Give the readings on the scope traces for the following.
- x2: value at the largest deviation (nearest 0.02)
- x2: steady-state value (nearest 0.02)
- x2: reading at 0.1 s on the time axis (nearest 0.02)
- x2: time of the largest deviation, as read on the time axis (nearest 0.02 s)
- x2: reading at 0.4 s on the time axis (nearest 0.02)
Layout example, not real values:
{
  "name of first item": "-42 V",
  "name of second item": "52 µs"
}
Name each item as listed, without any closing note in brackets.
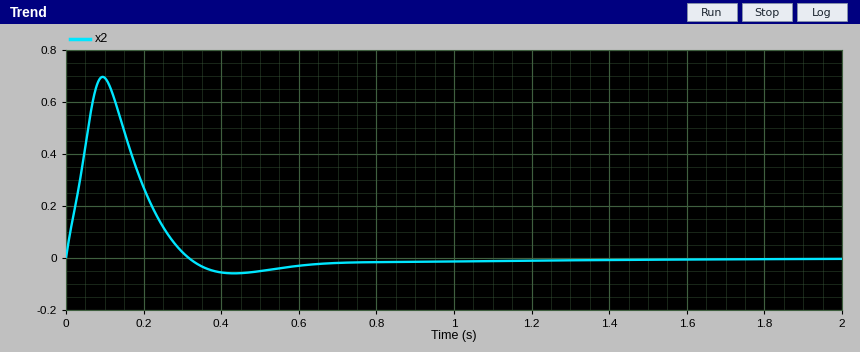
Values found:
{
  "x2: value at the largest deviation": "0.70",
  "x2: steady-state value": "0.00",
  "x2: reading at 0.1 s on the time axis": "0.70",
  "x2: time of the largest deviation, as read on the time axis": "0.10 s",
  "x2: reading at 0.4 s on the time axis": "-0.06"
}
